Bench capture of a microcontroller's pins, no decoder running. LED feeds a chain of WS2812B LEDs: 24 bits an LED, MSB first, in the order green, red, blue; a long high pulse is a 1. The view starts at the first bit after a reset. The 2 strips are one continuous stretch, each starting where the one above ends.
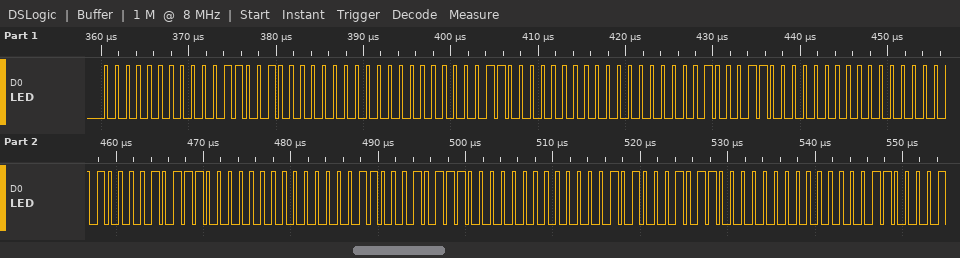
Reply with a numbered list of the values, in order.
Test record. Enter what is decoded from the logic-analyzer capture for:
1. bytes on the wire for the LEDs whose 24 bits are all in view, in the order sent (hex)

1. 00 19 00 00 18 00 01 18 00 02 17 00 03 17 00 05 16 00
